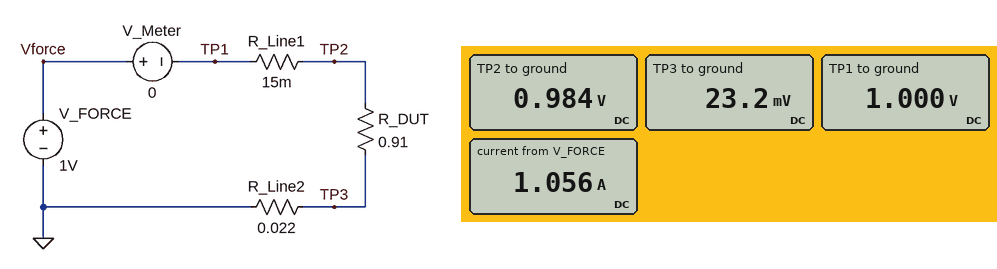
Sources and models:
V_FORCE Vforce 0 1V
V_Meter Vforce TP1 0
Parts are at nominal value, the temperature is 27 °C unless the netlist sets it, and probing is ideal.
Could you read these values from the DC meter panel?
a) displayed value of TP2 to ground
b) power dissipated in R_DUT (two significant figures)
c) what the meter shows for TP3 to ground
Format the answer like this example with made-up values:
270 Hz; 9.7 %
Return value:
0.984 V; 1.0 W; 23.2 mV
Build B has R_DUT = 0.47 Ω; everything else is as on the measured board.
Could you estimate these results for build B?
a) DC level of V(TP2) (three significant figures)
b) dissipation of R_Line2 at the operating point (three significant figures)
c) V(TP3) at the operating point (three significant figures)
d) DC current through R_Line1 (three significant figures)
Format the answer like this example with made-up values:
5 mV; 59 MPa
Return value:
970 mV; 85.6 mW; 43.4 mV; 1.97 A
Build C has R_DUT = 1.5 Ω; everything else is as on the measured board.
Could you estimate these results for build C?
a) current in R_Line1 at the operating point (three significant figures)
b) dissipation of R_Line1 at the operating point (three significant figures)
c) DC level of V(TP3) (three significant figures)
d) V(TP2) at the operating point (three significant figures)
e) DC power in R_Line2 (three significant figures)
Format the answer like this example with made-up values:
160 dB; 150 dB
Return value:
651 mA; 6.35 mW; 14.3 mV; 990 mV; 9.31 mW
